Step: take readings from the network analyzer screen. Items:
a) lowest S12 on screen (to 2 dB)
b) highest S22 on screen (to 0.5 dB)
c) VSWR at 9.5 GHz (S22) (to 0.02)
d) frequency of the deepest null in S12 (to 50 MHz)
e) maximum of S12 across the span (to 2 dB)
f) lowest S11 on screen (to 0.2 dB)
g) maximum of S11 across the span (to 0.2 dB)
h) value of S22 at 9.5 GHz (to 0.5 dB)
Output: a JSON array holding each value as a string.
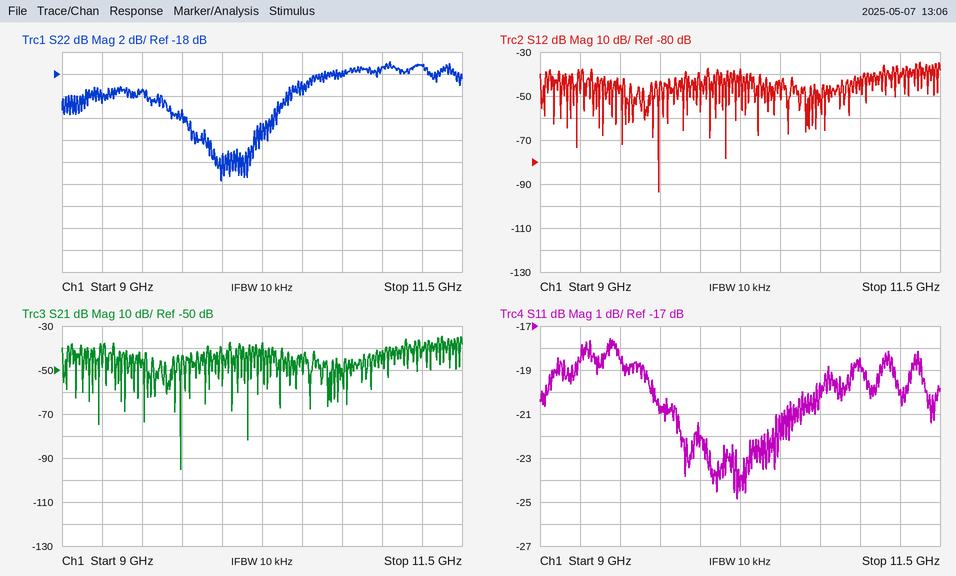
["-94 dB", "-17.0 dB", "1.24", "9.75 GHz", "-34 dB", "-24.8 dB", "-17.6 dB", "-19.5 dB"]
